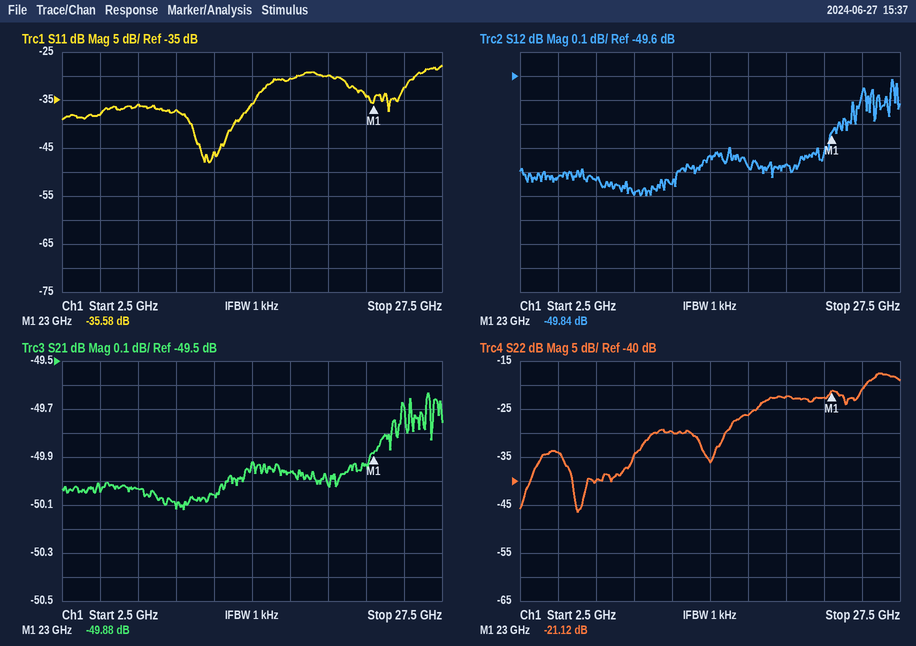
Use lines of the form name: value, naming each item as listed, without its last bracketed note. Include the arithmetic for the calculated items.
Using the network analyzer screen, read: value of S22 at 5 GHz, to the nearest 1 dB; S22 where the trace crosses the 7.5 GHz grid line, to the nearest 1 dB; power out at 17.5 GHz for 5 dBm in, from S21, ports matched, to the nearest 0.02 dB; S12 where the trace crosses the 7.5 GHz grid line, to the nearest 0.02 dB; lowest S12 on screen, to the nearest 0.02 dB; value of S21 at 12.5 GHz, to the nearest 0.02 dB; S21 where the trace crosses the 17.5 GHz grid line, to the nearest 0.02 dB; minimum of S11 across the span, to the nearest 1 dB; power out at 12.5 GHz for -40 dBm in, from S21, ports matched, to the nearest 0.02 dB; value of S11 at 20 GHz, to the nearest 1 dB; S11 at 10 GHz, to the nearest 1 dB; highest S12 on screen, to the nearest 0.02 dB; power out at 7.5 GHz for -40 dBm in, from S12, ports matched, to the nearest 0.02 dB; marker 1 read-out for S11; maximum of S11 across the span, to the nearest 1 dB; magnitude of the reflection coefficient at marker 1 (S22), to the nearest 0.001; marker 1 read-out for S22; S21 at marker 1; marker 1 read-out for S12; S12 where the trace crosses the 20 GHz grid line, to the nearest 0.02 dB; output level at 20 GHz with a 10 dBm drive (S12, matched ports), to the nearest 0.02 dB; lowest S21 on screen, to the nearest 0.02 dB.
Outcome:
value of S22 at 5 GHz, to the nearest 1 dB: -34 dB
S22 where the trace crosses the 7.5 GHz grid line, to the nearest 1 dB: -40 dB
power out at 17.5 GHz for 5 dBm in, from S21, ports matched, to the nearest 0.02 dB: 5 dBm + (-49.96 dB) = -44.96 dBm
S12 where the trace crosses the 7.5 GHz grid line, to the nearest 0.02 dB: -50.04 dB
lowest S12 on screen, to the nearest 0.02 dB: -50.10 dB
value of S21 at 12.5 GHz, to the nearest 0.02 dB: -50.06 dB
S21 where the trace crosses the 17.5 GHz grid line, to the nearest 0.02 dB: -49.96 dB
minimum of S11 across the span, to the nearest 1 dB: -48 dB
power out at 12.5 GHz for -40 dBm in, from S21, ports matched, to the nearest 0.02 dB: -40 dBm + (-50.06 dB) = -90.06 dBm
value of S11 at 20 GHz, to the nearest 1 dB: -30 dB
S11 at 10 GHz, to the nearest 1 dB: -37 dB
highest S12 on screen, to the nearest 0.02 dB: -49.62 dB
power out at 7.5 GHz for -40 dBm in, from S12, ports matched, to the nearest 0.02 dB: -40 dBm + (-50.04 dB) = -90.04 dBm
marker 1 read-out for S11: -35.58 dB
maximum of S11 across the span, to the nearest 1 dB: -28 dB
magnitude of the reflection coefficient at marker 1 (S22), to the nearest 0.001: 10^(-21.12/20) ≈ 0.088
marker 1 read-out for S22: -21.12 dB
S21 at marker 1: -49.88 dB
marker 1 read-out for S12: -49.84 dB
S12 where the trace crosses the 20 GHz grid line, to the nearest 0.02 dB: -49.96 dB
output level at 20 GHz with a 10 dBm drive (S12, matched ports), to the nearest 0.02 dB: 10 dBm + (-49.96 dB) = -39.96 dBm
lowest S21 on screen, to the nearest 0.02 dB: -50.12 dB
